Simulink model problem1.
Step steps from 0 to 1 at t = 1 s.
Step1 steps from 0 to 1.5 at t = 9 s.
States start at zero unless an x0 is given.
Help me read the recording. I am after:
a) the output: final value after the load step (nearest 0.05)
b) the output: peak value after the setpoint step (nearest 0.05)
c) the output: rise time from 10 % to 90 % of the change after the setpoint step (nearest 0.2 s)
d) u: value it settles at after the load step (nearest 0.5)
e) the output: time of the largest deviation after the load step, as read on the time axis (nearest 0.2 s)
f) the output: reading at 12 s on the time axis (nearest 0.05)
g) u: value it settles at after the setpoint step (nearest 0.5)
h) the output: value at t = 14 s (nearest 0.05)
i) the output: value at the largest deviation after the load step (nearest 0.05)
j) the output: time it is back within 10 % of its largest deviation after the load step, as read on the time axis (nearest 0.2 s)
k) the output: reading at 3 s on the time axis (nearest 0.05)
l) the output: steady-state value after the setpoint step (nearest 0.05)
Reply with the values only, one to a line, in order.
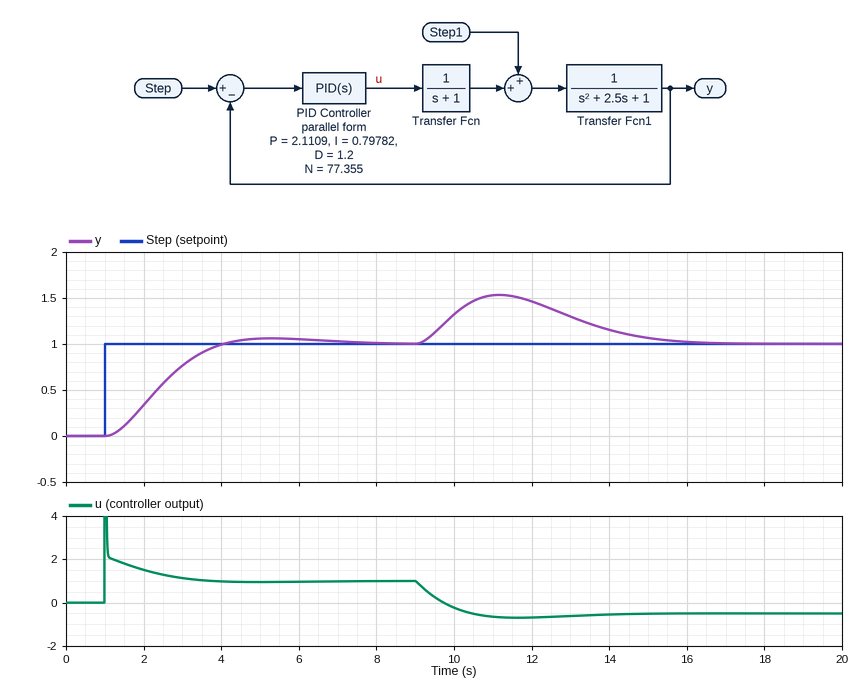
1.00
1.05
2.0 s
-0.5
11.2 s
1.45
1.0
1.15
1.55
15.2 s
0.75
1.00
